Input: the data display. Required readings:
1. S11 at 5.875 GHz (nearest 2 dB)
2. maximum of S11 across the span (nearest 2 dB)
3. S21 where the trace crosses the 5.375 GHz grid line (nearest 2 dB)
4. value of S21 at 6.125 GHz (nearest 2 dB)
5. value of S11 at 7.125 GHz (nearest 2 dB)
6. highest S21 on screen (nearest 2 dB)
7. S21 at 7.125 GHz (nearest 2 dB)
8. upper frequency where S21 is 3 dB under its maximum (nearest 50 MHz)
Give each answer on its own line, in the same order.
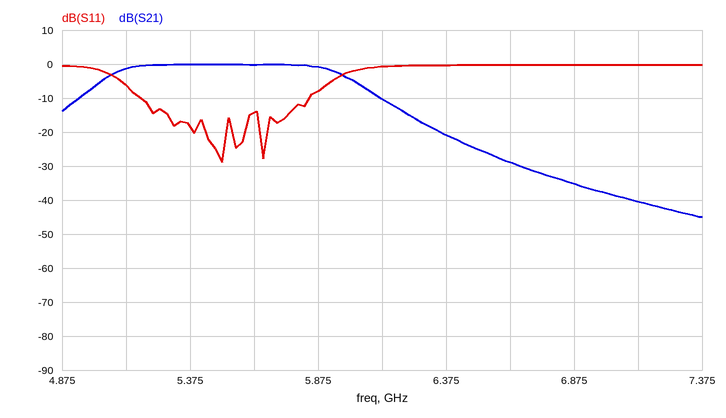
-8 dB
0 dB
0 dB
-10 dB
0 dB
0 dB
-40 dB
5.95 GHz
